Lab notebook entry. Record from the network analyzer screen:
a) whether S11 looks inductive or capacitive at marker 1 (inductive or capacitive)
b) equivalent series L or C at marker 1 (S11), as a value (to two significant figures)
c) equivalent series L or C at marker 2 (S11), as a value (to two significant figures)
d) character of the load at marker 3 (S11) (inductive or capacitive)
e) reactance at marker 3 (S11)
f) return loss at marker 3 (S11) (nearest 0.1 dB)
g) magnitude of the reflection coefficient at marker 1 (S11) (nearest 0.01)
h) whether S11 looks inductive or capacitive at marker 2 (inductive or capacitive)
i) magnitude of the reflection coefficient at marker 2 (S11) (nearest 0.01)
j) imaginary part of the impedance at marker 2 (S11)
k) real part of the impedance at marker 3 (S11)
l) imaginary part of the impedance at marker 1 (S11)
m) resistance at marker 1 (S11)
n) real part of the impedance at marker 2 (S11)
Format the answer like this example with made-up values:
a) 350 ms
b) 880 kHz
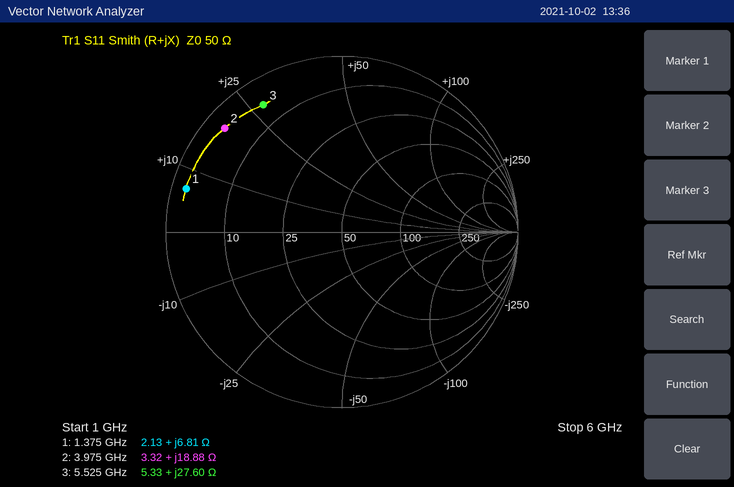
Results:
a) inductive
b) 790 pH
c) 760 pH
d) inductive
e) +27.60 Ω
f) 1.4 dB
g) 0.92
h) inductive
i) 0.89
j) +18.88 Ω
k) 5.33 Ω
l) +6.81 Ω
m) 2.13 Ω
n) 3.32 Ω
